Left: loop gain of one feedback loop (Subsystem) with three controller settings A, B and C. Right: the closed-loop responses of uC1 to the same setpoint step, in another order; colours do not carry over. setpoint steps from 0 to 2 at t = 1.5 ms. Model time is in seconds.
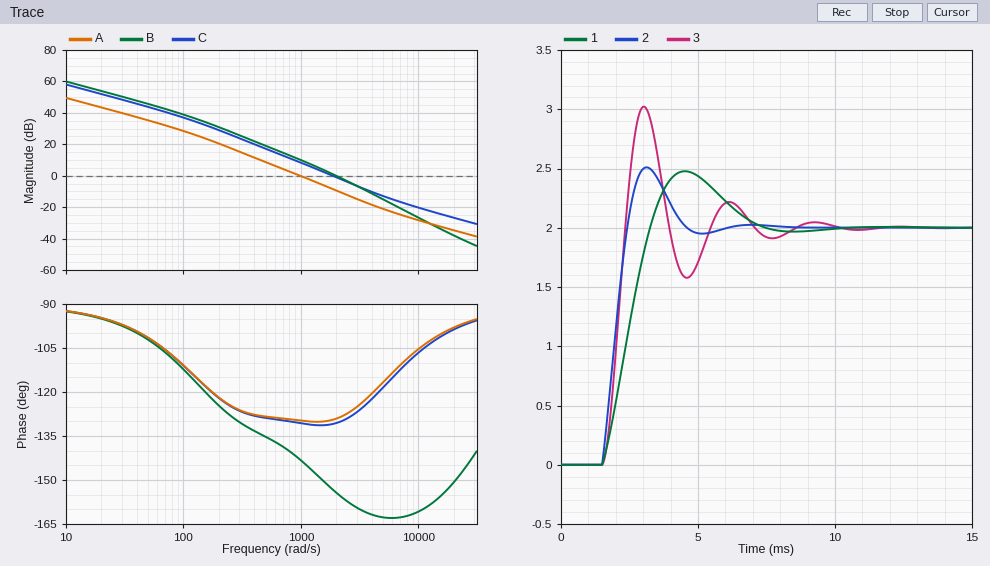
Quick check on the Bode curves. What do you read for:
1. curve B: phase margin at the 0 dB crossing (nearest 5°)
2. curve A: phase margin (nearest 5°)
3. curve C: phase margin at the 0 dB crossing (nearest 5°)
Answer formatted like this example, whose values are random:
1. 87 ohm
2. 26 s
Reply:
1. 25°
2. 50°
3. 50°
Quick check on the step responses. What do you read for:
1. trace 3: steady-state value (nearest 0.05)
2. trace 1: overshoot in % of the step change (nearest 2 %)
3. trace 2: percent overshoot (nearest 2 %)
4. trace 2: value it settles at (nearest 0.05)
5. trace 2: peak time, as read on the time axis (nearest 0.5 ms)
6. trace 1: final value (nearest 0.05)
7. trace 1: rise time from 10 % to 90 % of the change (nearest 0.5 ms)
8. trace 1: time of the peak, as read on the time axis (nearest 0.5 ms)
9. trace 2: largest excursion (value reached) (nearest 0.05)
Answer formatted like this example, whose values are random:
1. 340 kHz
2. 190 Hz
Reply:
1. 2.00
2. 24 %
3. 26 %
4. 2.00
5. 3.0 ms
6. 2.00
7. 1.5 ms
8. 4.5 ms
9. 2.50
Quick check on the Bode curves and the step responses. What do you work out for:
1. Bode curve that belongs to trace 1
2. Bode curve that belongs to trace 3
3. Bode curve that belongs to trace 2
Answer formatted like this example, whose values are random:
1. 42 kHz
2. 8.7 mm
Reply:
1. A
2. B
3. C
